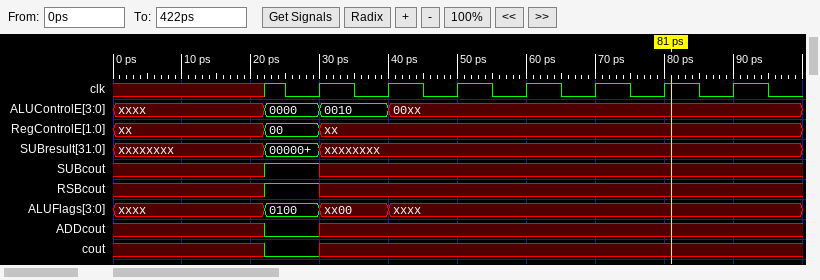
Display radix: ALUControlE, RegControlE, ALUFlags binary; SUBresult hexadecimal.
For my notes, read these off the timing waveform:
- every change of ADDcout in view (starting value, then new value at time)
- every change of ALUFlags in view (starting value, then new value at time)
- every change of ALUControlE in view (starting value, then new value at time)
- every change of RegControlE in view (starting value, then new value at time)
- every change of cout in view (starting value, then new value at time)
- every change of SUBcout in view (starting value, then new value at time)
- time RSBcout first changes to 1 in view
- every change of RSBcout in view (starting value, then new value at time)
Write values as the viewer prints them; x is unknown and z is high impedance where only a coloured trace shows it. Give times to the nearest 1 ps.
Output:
x, 0 at 22 ps, x at 30 ps
xxxx, 0100 at 22 ps, xx00 at 30 ps, xxxx at 40 ps
xxxx, 0000 at 22 ps, 0010 at 30 ps, 00xx at 40 ps
xx, 00 at 22 ps, xx at 30 ps
x, 0 at 22 ps, x at 30 ps
x, 1 at 22 ps, x at 30 ps
22 ps
x, 1 at 22 ps, x at 30 ps
